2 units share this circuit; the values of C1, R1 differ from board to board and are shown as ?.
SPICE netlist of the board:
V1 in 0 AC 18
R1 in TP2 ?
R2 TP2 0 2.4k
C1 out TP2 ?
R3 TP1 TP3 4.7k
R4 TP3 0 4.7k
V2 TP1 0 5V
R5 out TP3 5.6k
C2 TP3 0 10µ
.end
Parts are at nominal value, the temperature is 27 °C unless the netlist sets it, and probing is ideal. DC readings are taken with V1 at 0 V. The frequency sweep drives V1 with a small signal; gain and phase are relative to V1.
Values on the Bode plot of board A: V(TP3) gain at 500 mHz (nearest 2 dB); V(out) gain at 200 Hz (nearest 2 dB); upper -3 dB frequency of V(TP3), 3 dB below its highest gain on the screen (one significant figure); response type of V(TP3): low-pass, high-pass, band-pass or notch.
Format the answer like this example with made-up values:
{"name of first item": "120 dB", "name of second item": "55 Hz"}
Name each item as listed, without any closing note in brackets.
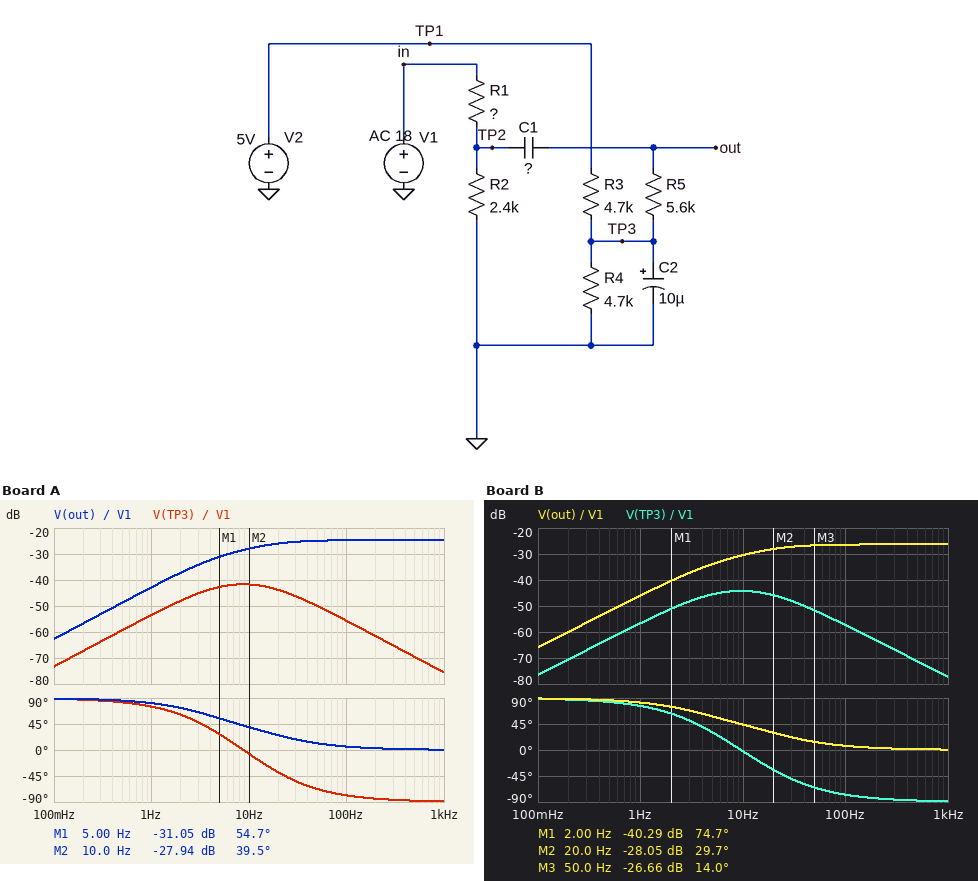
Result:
{"V(TP3) gain at 500 mHz": "-60 dB", "V(out) gain at 200 Hz": "-24 dB", "upper -3 dB frequency of V(TP3), 3 dB below its highest gain on the screen": "20 Hz", "response type of V(TP3): low-pass, high-pass, band-pass or notch": "band-pass"}
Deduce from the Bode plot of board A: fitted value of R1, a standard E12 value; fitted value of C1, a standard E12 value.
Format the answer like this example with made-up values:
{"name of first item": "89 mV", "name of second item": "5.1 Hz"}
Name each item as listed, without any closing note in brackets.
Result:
{"fitted value of R1, a standard E12 value": "27 kΩ", "fitted value of C1, a standard E12 value": "1.8 µF"}
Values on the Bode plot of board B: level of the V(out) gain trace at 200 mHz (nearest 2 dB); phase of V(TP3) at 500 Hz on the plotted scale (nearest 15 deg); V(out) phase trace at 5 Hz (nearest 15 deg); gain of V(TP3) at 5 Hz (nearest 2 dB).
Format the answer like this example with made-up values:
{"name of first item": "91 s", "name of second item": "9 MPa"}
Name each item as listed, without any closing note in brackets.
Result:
{"level of the V(out) gain trace at 200 mHz": "-60 dB", "phase of V(TP3) at 500 Hz on the plotted scale": "-90 deg", "V(out) phase trace at 5 Hz": "60 deg", "gain of V(TP3) at 5 Hz": "-46 dB"}
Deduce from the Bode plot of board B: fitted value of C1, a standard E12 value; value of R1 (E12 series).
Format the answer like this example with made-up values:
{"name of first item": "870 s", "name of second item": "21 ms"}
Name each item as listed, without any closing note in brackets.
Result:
{"fitted value of C1, a standard E12 value": "1.5 µF", "value of R1": "33 kΩ"}
